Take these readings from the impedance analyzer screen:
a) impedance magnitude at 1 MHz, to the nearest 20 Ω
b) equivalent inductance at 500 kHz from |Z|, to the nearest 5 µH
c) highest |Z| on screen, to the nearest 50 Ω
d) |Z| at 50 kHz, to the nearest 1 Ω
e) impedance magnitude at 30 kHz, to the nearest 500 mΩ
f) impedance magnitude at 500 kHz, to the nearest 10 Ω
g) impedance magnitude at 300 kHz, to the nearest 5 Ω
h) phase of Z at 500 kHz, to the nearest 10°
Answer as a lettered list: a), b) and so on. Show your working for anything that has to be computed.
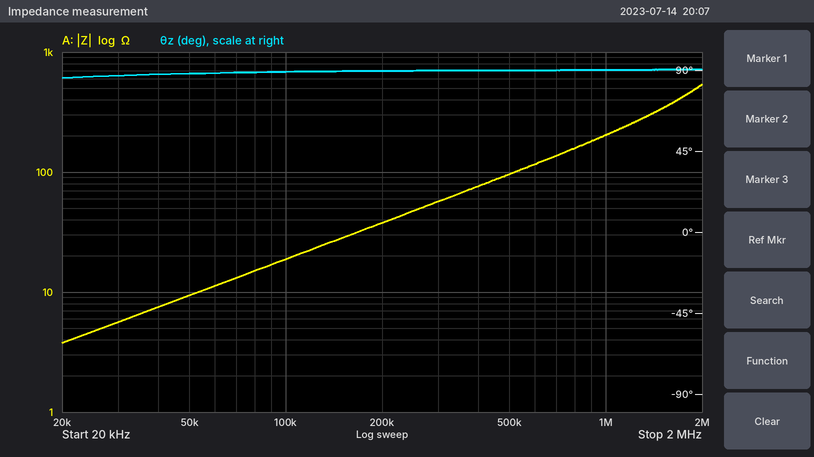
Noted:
a) 200 Ω
b) L = 100 Ω/(2π × 500 kHz) ≈ 31.8 µH, so 30 µH to the nearest 5 µH
c) 550 Ω
d) 9 Ω
e) 5.5 Ω
f) 100 Ω
g) 55 Ω
h) 90°
